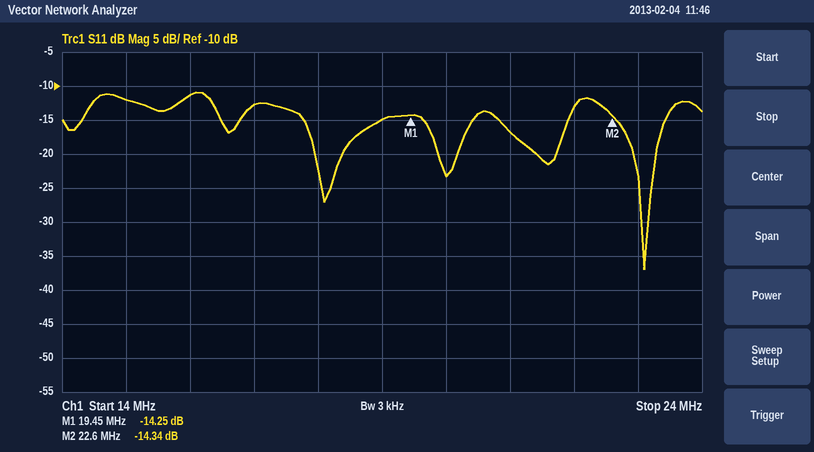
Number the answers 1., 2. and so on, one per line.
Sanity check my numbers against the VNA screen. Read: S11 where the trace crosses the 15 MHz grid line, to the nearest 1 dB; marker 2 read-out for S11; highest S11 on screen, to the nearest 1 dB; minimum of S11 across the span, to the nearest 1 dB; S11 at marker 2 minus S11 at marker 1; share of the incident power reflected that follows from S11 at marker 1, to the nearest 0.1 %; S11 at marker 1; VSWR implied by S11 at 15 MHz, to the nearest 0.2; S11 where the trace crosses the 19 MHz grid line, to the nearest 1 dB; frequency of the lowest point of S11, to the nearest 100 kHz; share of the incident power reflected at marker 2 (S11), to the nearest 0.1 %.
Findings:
1. -12 dB
2. -14.34 dB
3. -11 dB
4. -37 dB
5. -0.09 dB
6. 3.8 %
7. -14.25 dB
8. 1.6
9. -15 dB
10. 23.1 MHz
11. 3.7 %
